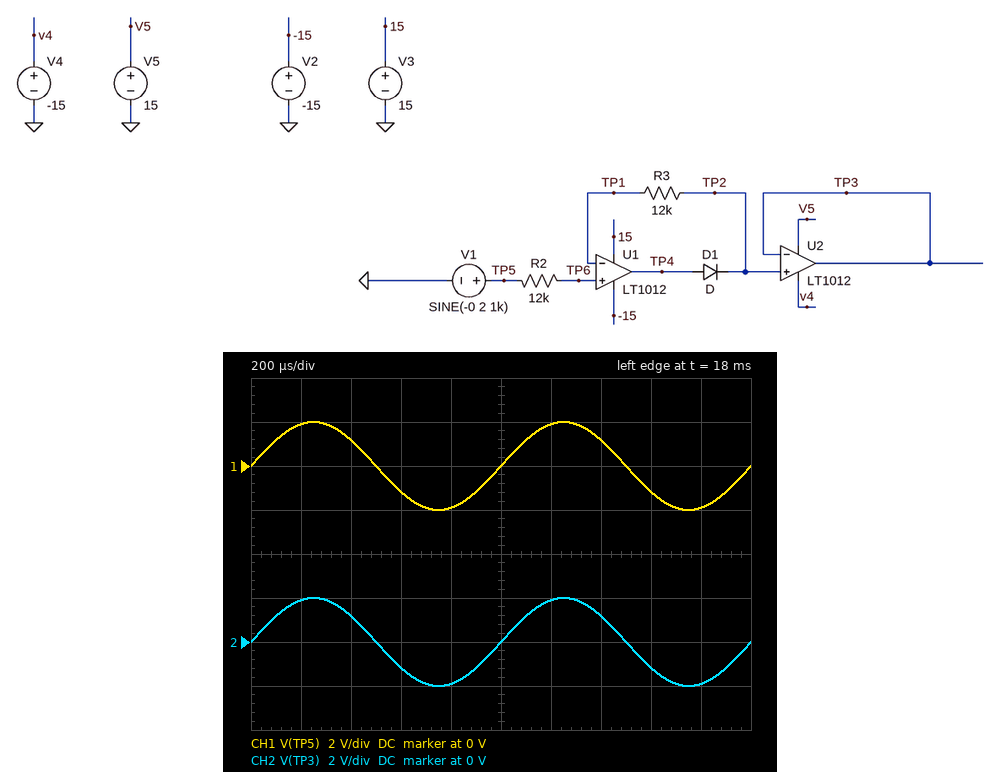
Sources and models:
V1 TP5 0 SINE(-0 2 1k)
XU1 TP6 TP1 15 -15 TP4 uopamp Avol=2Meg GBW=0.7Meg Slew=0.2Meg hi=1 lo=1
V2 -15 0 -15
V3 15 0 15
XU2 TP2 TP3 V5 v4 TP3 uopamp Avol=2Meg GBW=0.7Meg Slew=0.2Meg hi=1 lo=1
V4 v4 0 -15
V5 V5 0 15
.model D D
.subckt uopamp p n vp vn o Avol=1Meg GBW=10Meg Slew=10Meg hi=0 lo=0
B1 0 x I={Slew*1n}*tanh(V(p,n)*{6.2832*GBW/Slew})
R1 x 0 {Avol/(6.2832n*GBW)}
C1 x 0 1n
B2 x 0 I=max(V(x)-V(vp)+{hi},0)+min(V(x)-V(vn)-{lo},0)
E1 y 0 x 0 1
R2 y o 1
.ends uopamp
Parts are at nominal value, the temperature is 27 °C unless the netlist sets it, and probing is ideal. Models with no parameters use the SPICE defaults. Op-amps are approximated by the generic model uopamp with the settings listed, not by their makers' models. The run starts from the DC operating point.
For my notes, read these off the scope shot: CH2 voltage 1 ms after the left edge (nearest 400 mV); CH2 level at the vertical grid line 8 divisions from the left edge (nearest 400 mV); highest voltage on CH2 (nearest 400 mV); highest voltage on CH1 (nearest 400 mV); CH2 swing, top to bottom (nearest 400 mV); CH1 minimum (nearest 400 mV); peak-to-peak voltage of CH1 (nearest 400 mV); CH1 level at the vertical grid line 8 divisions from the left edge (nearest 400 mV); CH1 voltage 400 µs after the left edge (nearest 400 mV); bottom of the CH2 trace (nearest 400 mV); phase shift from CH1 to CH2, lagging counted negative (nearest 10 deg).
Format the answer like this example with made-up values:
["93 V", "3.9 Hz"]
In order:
["0 V", "-1.2 V", "2.0 V", "2.0 V", "4.0 V", "-2.0 V", "4.0 V", "-1.2 V", "1.2 V", "-2.0 V", "0 deg"]
